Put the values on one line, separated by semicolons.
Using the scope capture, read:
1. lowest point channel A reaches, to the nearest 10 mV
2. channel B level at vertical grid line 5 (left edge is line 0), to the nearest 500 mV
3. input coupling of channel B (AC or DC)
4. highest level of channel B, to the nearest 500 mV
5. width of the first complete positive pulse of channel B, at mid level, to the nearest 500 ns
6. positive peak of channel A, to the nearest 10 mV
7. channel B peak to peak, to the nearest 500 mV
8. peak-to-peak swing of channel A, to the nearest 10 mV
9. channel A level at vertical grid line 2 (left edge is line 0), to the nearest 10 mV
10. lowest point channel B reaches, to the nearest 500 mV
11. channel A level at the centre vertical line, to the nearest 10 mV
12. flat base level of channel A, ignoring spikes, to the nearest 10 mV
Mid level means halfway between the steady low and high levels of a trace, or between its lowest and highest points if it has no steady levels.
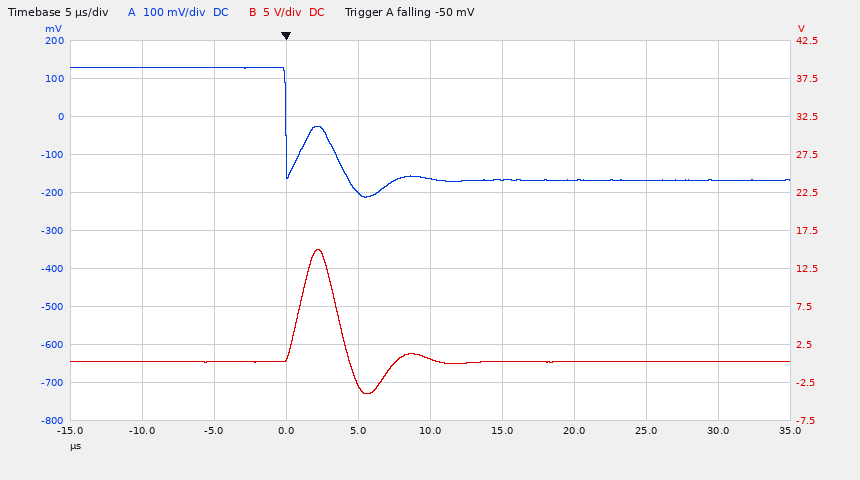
-210 mV; 500 mV; DC; 15.0 V; 3.0 µs; 130 mV; 19.0 V; 340 mV; 130 mV; -4.0 V; -160 mV; -170 mV
